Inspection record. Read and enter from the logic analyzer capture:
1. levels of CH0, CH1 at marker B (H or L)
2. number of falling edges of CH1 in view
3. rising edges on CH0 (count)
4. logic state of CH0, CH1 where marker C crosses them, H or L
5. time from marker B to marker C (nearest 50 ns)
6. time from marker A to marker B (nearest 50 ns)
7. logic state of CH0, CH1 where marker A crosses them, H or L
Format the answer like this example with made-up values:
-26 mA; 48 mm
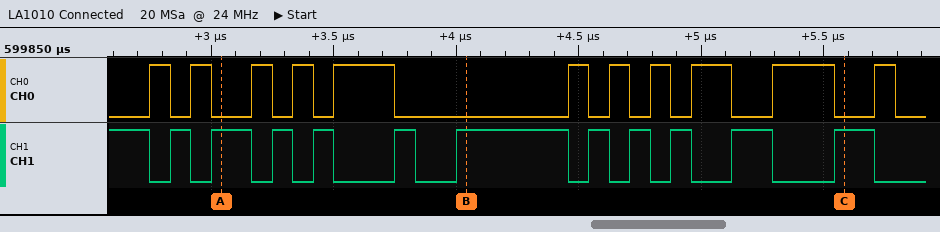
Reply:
CH0=L, CH1=H; 12; 11; CH0=L, CH1=H; 1550 ns; 1000 ns; CH0=L, CH1=H
